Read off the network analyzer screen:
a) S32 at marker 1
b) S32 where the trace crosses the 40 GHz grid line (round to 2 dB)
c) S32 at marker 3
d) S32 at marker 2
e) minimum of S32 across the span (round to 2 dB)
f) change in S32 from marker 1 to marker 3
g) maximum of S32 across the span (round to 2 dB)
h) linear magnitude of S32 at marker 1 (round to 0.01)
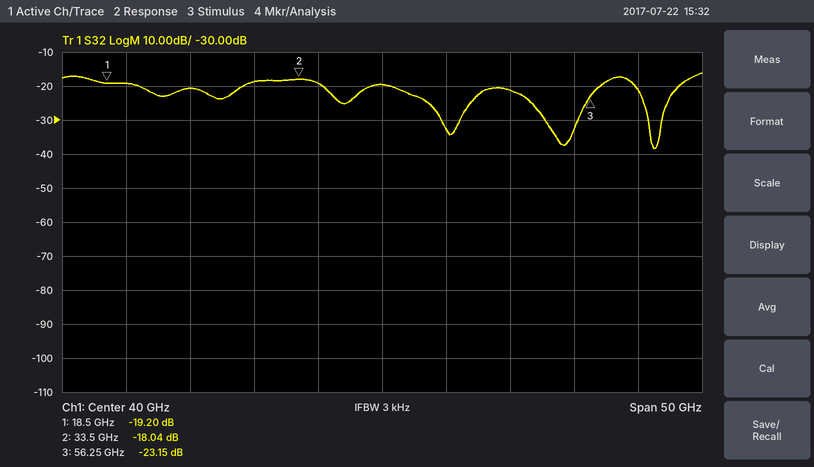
-19.20 dB
-20 dB
-23.15 dB
-18.04 dB
-38 dB
-3.95 dB
-16 dB
0.11
